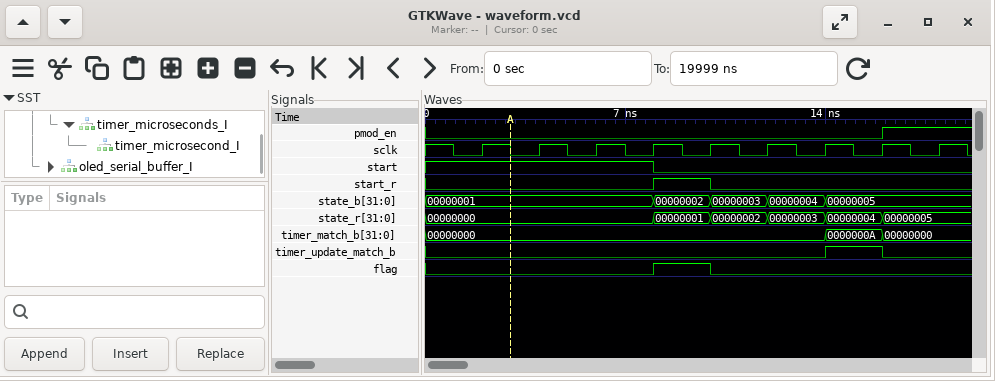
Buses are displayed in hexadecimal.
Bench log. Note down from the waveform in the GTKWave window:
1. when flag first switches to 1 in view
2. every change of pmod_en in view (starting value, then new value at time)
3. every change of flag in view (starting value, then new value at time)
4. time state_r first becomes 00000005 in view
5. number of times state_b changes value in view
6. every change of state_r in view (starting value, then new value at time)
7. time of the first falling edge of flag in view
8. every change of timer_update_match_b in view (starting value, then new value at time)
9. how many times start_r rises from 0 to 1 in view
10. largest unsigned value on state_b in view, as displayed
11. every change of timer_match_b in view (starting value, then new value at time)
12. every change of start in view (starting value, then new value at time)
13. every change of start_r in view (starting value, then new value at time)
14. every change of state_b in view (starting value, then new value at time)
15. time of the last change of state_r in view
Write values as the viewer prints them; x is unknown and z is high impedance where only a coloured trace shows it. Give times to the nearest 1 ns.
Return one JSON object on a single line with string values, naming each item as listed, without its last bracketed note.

{"when flag first switches to 1 in view": "8 ns", "every change of pmod_en in view": "0, 1 at 16 ns", "every change of flag in view": "0, 1 at 8 ns, 0 at 10 ns", "time state_r first becomes 00000005 in view": "16 ns", "number of times state_b changes value in view": "4", "every change of state_r in view": "00000000, 00000001 at 8 ns, 00000002 at 10 ns, 00000003 at 12 ns, 00000004 at 14 ns, 00000005 at 16 ns", "time of the first falling edge of flag in view": "10 ns", "every change of timer_update_match_b in view": "0, 1 at 14 ns, 0 at 16 ns", "how many times start_r rises from 0 to 1 in view": "1", "largest unsigned value on state_b in view, as displayed": "00000005", "every change of timer_match_b in view": "00000000, 0000000A at 14 ns, 00000000 at 16 ns", "every change of start in view": "1, 0 at 8 ns", "every change of start_r in view": "0, 1 at 8 ns, 0 at 10 ns", "every change of state_b in view": "00000001, 00000002 at 8 ns, 00000003 at 10 ns, 00000004 at 12 ns, 00000005 at 14 ns", "time of the last change of state_r in view": "16 ns"}
